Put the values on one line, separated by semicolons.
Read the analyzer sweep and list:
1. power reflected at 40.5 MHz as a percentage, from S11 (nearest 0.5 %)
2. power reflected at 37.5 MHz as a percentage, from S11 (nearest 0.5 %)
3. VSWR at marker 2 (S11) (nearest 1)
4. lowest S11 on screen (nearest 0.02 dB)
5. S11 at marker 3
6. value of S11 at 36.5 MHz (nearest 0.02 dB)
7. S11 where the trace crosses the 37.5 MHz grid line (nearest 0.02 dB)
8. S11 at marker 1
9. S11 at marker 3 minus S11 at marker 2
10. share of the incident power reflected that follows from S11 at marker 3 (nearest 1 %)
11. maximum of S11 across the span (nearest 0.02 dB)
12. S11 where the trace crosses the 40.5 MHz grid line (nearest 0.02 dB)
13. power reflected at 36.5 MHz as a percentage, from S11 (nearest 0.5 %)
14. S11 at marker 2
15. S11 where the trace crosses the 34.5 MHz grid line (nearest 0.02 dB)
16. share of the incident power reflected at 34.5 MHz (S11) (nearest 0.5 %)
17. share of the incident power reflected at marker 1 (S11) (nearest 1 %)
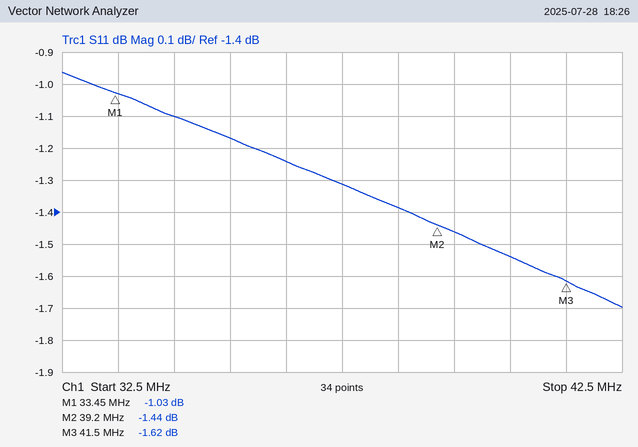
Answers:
70.0 %; 74.0 %; 12; -1.70 dB; -1.62 dB; -1.24 dB; -1.32 dB; -1.03 dB; -0.18 dB; 69 %; -0.96 dB; -1.54 dB; 75.0 %; -1.44 dB; -1.10 dB; 77.5 %; 79 %
